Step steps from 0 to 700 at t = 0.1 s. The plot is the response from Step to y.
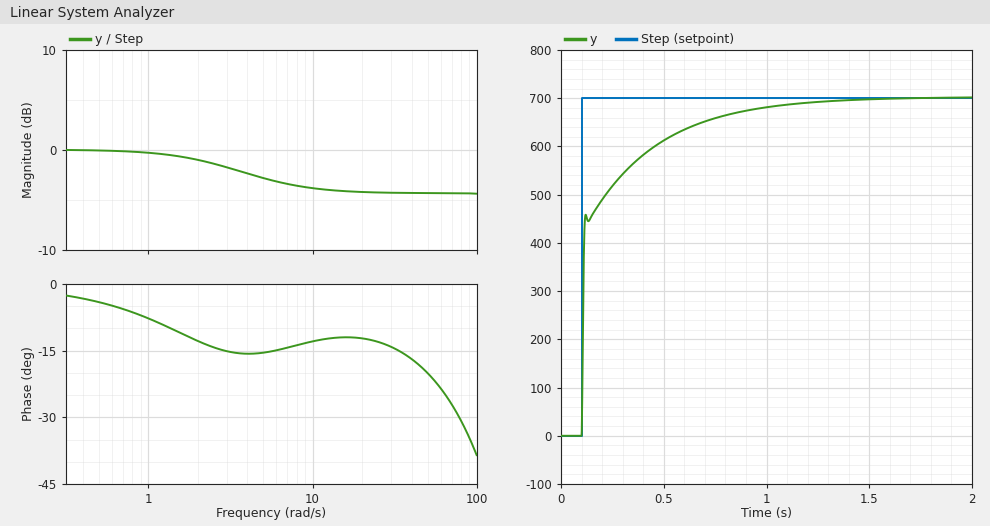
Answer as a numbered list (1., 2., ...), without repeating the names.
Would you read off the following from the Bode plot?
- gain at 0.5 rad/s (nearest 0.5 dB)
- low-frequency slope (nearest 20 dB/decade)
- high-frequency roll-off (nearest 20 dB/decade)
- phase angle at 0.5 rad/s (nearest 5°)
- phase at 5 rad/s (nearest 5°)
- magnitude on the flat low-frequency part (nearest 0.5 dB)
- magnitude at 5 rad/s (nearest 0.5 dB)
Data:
1. 0.0 dB
2. 0 dB/decade
3. 0 dB/decade
4. -5°
5. -15°
6. 0.0 dB
7. -3.0 dB
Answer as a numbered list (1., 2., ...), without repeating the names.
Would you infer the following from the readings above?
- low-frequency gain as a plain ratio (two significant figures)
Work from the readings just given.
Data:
1. 1.0
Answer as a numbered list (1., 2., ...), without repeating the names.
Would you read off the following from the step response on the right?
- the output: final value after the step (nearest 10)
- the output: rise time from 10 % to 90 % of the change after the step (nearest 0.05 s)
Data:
1. 700
2. 0.50 s
